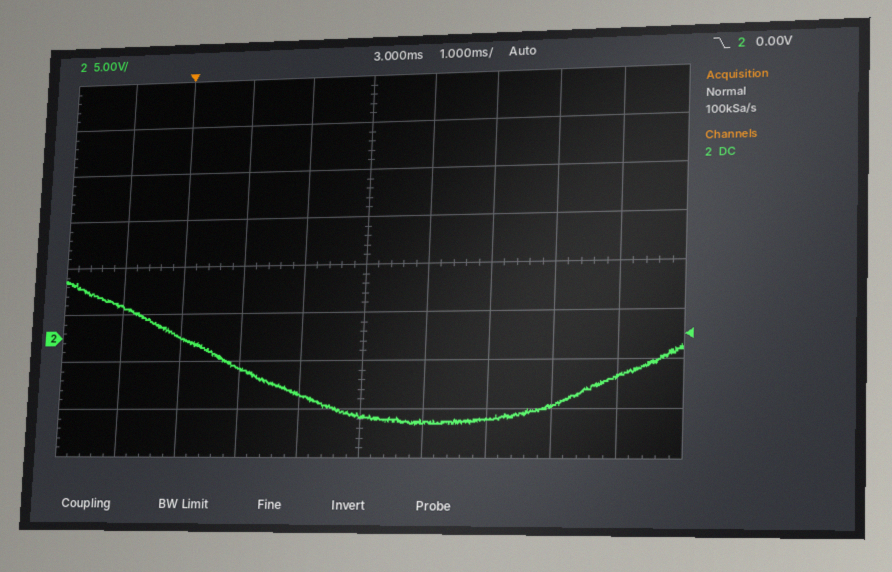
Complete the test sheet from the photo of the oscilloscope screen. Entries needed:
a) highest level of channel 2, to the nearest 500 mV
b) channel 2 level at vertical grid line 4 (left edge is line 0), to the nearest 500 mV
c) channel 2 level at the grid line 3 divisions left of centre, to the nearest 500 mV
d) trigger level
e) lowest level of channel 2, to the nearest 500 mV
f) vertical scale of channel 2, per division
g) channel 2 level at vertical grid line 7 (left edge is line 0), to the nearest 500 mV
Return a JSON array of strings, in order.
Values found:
["6.0 V", "-6.0 V", "0.0 V", "0.00 V", "-9.0 V", "5 V", "-8.5 V"]
